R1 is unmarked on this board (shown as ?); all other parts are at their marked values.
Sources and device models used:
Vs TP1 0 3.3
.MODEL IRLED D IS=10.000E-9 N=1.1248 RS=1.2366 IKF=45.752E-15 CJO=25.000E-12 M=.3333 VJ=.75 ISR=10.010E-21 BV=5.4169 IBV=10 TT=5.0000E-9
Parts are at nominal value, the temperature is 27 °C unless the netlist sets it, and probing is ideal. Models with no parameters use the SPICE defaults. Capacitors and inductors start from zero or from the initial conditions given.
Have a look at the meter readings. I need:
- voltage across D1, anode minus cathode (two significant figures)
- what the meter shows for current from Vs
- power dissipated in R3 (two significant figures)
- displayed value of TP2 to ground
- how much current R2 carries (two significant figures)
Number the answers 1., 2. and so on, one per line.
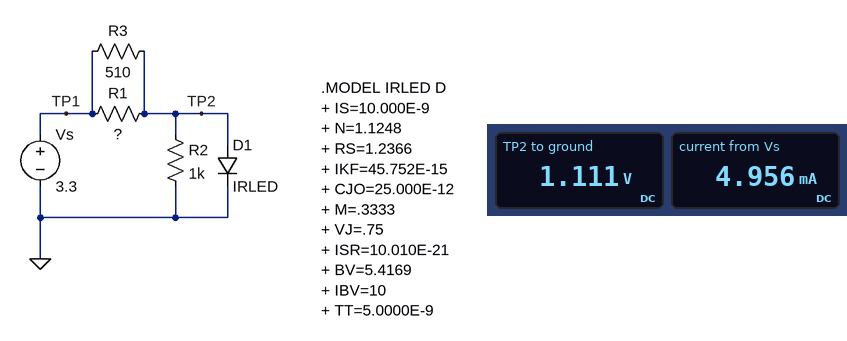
1. 1.1 V
2. 4.956 mA
3. 9.4 mW
4. 1.111 V
5. 1.1 mA
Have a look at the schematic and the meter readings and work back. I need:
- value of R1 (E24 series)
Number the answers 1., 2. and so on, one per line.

1. 3.3 kΩ
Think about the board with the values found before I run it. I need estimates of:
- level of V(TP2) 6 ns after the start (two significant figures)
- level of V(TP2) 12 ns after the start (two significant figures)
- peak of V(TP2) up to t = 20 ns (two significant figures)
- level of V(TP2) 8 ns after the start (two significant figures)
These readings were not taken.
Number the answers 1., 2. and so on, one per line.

1. 940 mV
2. 1.1 V
3. 1.1 V
4. 1.0 V
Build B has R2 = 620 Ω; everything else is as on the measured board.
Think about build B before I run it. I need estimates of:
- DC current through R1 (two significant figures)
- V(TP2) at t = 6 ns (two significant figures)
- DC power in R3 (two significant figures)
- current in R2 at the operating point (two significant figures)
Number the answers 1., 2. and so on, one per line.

1. 670 µA
2. 910 mV
3. 9.5 mW
4. 1.8 mA
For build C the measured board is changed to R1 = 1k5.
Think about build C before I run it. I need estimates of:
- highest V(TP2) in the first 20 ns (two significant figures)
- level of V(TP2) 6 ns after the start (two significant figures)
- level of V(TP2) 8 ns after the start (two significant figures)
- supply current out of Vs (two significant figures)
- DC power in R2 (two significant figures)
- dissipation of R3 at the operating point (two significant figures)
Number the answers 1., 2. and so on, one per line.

1. 1.1 V
2. 1.0 V
3. 1.1 V
4. 5.7 mA
5. 1.3 mW
6. 9.3 mW
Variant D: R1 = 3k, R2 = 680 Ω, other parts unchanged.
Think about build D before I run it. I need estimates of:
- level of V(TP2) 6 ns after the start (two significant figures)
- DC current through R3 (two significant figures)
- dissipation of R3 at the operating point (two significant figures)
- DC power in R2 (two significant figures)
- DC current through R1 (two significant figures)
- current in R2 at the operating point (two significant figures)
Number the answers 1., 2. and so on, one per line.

1. 920 mV
2. 4.3 mA
3. 9.5 mW
4. 1.8 mW
5. 730 µA
6. 1.6 mA
